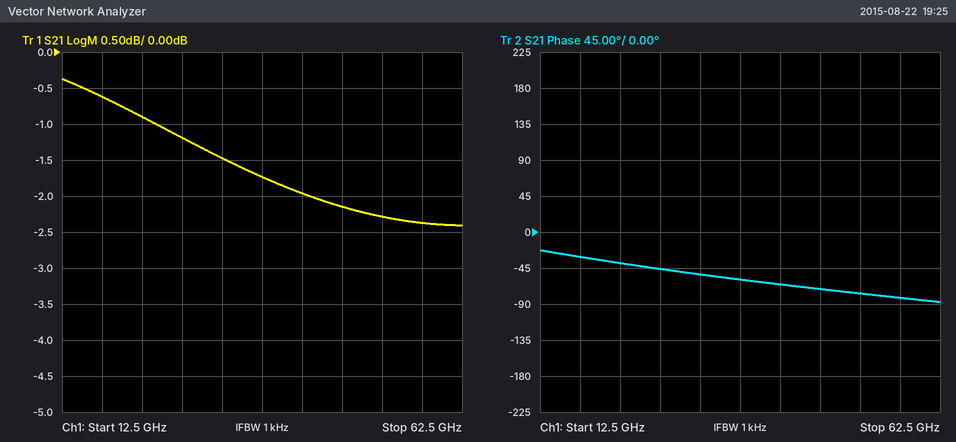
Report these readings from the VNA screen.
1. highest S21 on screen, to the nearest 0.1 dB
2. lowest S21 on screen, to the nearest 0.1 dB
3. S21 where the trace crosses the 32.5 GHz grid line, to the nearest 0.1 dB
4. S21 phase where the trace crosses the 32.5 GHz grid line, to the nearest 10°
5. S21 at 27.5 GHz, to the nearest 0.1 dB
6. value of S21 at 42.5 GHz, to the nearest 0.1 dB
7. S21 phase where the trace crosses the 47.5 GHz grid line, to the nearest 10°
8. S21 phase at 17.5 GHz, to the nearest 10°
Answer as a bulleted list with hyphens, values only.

- -0.4 dB
- -2.4 dB
- -1.5 dB
- -50°
- -1.2 dB
- -2.0 dB
- -70°
- -30°
